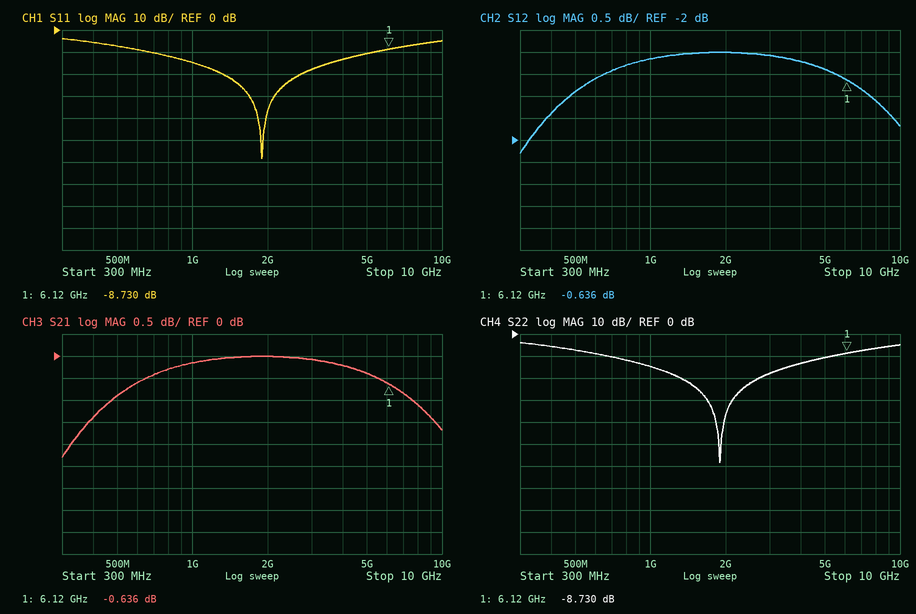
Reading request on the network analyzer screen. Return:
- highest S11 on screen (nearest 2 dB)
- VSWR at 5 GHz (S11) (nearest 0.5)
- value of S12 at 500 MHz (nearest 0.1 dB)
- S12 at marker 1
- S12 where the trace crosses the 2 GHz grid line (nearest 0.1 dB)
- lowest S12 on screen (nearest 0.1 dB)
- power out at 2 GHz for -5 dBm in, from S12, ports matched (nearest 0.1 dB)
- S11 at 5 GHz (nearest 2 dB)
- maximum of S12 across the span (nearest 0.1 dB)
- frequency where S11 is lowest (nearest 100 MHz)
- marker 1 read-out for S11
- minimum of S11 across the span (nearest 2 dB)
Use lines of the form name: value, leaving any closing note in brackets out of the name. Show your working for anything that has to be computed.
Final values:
highest S11 on screen: -4 dB
VSWR at 5 GHz (S11): |Γ| = 10^(-10/20) = 0.3162; VSWR = (1 + 0.3162)/(1 − 0.3162) ≈ 1.92, so 2.0 to the nearest 0.5
value of S12 at 500 MHz: -0.9 dB
S12 at marker 1: -0.636 dB
S12 where the trace crosses the 2 GHz grid line: 0.0 dB
lowest S12 on screen: -2.3 dB
power out at 2 GHz for -5 dBm in, from S12, ports matched: -5 dBm + (0.0 dB) = -5.0 dBm
S11 at 5 GHz: -10 dB
maximum of S12 across the span: 0.0 dB
frequency where S11 is lowest: 1.9 GHz
marker 1 read-out for S11: -8.730 dB
minimum of S11 across the span: -58 dB
